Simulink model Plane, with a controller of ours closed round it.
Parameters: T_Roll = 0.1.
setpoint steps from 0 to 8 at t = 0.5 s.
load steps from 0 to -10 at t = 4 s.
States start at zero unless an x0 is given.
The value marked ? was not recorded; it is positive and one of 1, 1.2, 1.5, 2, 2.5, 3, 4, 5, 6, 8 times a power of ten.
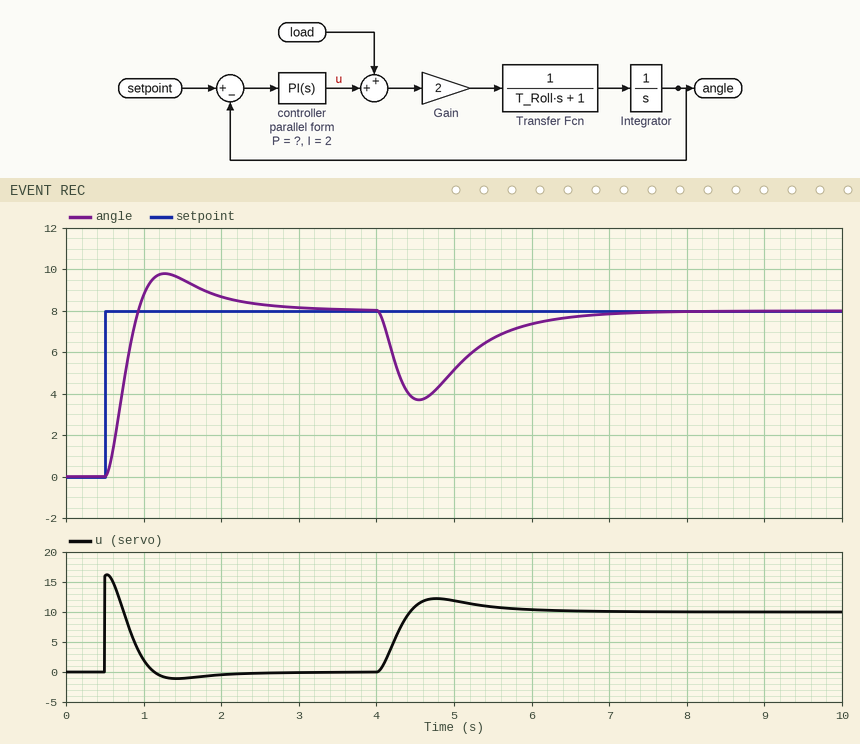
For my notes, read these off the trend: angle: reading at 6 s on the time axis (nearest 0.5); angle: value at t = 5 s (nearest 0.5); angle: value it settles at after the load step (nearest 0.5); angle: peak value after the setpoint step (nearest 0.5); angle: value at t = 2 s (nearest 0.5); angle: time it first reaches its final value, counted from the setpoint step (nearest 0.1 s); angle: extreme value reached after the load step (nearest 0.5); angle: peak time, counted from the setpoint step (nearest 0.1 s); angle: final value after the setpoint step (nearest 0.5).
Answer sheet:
7.5
5.0
8.0
10.0
8.5
0.4 s
3.5
0.8 s
8.0
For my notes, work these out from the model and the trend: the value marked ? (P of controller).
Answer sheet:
2
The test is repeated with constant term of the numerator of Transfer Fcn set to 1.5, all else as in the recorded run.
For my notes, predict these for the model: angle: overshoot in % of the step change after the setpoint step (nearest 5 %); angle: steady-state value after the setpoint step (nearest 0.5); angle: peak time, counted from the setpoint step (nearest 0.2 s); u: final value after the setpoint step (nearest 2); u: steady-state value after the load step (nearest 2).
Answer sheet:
25 %
8.0
0.6 s
0
10
